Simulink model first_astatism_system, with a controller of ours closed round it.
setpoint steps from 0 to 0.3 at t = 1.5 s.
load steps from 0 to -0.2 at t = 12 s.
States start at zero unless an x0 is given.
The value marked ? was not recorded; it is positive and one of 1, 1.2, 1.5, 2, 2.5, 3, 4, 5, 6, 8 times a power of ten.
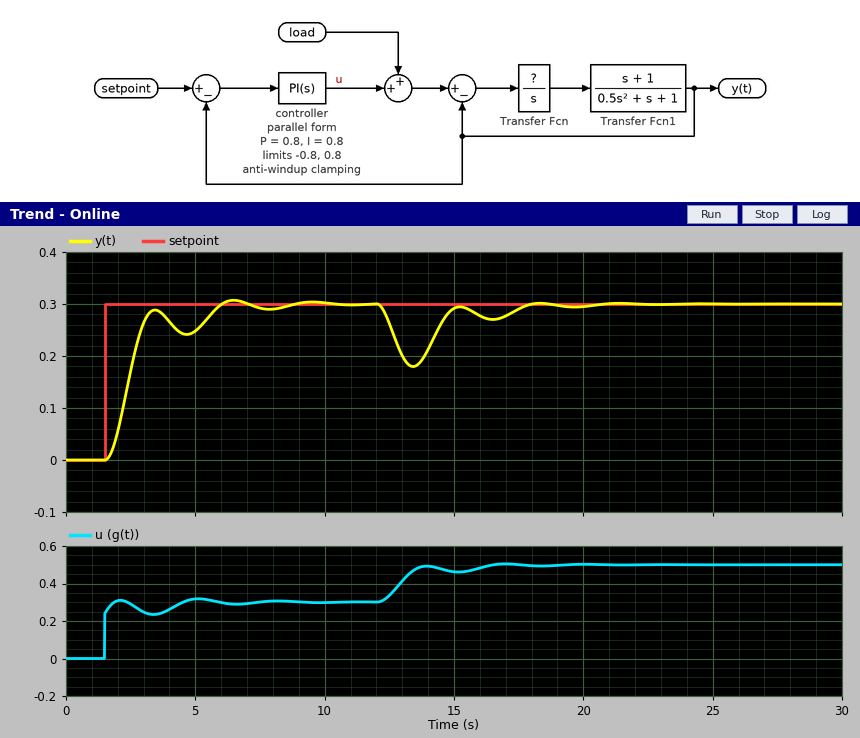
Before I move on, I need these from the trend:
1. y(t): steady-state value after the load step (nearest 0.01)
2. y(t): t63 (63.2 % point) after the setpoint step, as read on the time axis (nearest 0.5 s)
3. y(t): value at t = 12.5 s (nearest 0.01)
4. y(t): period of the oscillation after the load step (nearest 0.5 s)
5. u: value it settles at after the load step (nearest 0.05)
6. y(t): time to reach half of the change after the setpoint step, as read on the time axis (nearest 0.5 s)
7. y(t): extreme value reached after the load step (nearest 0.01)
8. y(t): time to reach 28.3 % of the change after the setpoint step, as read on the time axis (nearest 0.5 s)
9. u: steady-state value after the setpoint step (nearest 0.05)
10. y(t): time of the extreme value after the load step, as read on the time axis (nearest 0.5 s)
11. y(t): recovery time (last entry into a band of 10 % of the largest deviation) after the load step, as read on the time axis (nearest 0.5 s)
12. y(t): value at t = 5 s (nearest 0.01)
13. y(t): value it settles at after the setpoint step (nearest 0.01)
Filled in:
0.30
2.5 s
0.26
3.0 s
0.50
2.5 s
0.18
2.0 s
0.30
13.5 s
17.5 s
0.25
0.30
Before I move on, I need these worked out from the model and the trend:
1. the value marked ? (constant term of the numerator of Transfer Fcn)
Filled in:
1
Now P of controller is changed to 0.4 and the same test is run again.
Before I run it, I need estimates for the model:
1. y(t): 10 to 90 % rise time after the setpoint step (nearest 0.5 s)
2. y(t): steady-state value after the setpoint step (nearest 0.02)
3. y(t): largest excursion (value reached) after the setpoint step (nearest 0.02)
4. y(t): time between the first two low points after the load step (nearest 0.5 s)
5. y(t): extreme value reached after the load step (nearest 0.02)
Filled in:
1.5 s
0.30
0.32
3.5 s
0.16
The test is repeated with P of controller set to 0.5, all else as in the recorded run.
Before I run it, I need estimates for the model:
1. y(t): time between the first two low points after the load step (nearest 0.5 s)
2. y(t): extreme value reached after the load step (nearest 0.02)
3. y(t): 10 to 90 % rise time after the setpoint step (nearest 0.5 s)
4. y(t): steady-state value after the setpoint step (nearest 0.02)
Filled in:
3.5 s
0.16
1.5 s
0.30
